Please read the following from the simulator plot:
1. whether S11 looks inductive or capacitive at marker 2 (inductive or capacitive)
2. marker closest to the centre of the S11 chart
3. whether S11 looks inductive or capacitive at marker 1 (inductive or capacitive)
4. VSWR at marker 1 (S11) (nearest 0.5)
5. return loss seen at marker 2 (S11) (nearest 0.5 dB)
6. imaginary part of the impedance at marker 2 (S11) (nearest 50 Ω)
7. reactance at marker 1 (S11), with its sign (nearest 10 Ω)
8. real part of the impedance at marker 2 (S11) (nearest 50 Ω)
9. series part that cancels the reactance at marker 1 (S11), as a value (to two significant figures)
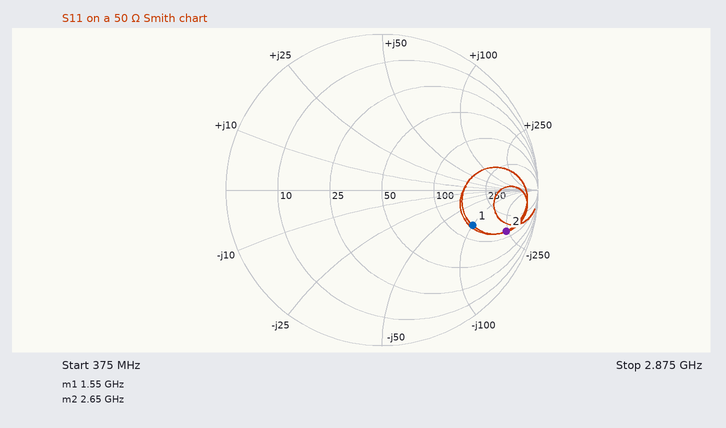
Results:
capacitive
marker 1
capacitive
4.5
1.5 dB
-250 Ω
-100 Ω
150 Ω
10 nH
